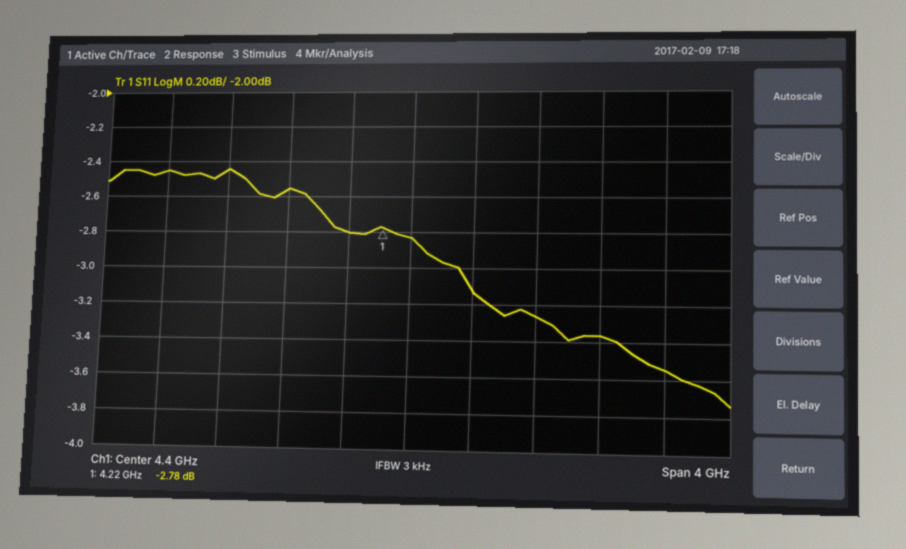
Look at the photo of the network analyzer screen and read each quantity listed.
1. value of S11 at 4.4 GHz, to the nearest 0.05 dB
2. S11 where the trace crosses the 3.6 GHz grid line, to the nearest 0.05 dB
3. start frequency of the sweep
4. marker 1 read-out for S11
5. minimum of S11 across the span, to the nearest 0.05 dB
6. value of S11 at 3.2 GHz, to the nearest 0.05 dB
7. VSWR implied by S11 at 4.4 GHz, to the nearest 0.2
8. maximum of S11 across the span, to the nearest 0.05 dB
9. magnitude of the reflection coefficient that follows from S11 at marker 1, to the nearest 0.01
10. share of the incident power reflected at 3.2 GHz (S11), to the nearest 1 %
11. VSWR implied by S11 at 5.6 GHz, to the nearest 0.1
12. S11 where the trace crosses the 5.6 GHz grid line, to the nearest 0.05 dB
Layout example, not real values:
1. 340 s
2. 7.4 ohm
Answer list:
1. -2.85 dB
2. -2.55 dB
3. 2.4 GHz
4. -2.78 dB
5. -3.75 dB
6. -2.45 dB
7. 6.2
8. -2.45 dB
9. 0.73
10. 57 %
11. 5.2
12. -3.35 dB
